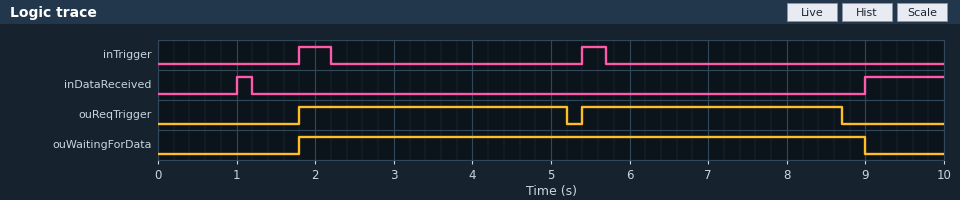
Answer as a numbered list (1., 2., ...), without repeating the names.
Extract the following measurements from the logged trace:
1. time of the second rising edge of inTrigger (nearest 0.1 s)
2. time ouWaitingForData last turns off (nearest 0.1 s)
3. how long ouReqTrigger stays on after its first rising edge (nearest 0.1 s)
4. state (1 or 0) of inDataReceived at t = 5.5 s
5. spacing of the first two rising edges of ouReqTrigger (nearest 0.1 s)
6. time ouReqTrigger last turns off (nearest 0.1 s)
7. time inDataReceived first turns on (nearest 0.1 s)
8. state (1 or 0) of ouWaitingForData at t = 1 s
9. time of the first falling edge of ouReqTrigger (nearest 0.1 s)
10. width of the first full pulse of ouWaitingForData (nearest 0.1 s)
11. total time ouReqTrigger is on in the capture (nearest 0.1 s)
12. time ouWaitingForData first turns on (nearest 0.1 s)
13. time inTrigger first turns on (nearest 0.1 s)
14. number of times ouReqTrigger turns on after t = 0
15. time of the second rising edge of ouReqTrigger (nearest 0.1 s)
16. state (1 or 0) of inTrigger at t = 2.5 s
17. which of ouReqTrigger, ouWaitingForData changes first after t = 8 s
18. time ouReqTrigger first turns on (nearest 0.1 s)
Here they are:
1. 5.4 s
2. 9.0 s
3. 3.4 s
4. 0
5. 3.6 s
6. 8.7 s
7. 1.0 s
8. 0
9. 5.2 s
10. 7.2 s
11. 6.7 s
12. 1.8 s
13. 1.8 s
14. 2
15. 5.4 s
16. 0
17. ouReqTrigger
18. 1.8 s
